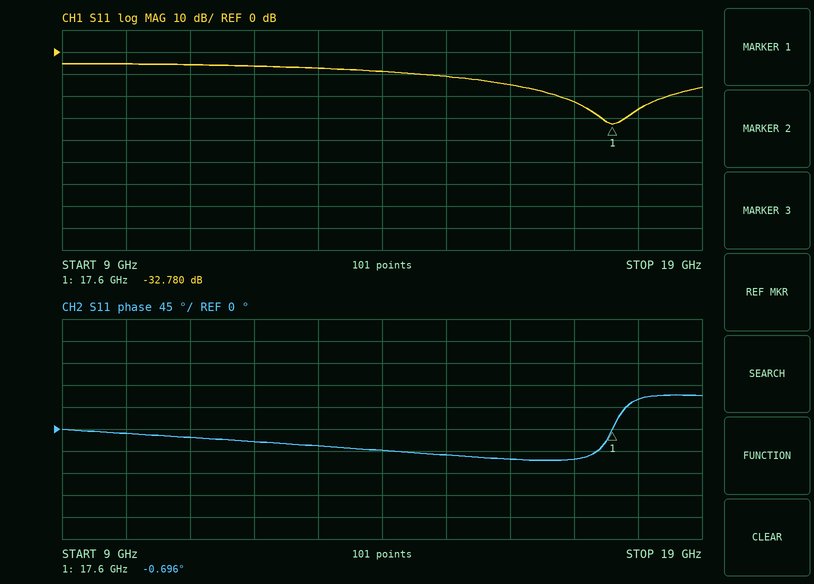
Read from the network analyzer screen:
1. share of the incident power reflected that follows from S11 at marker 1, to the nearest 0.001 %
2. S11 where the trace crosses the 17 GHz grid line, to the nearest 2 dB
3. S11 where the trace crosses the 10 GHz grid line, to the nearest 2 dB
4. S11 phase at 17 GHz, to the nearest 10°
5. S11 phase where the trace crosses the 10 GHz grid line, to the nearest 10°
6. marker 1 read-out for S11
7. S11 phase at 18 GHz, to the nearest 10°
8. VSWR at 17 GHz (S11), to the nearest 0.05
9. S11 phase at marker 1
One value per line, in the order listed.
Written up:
0.053 %
-22 dB
-6 dB
-60°
-10°
-32.780 dB
60°
1.15
-0.696°
